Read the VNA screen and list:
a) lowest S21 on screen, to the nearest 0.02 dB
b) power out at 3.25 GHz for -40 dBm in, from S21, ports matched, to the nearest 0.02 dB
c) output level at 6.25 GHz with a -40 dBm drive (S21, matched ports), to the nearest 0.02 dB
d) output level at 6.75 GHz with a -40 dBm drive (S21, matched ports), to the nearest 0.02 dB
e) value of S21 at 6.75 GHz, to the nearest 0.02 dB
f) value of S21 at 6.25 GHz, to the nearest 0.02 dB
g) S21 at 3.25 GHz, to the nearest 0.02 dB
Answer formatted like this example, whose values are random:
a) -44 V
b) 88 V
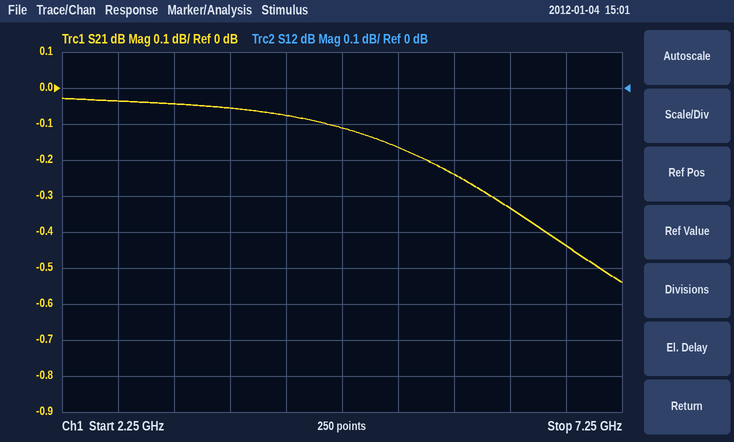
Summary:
a) -0.54 dB
b) -40.04 dBm
c) -40.34 dBm
d) -40.44 dBm
e) -0.44 dB
f) -0.34 dB
g) -0.04 dB
